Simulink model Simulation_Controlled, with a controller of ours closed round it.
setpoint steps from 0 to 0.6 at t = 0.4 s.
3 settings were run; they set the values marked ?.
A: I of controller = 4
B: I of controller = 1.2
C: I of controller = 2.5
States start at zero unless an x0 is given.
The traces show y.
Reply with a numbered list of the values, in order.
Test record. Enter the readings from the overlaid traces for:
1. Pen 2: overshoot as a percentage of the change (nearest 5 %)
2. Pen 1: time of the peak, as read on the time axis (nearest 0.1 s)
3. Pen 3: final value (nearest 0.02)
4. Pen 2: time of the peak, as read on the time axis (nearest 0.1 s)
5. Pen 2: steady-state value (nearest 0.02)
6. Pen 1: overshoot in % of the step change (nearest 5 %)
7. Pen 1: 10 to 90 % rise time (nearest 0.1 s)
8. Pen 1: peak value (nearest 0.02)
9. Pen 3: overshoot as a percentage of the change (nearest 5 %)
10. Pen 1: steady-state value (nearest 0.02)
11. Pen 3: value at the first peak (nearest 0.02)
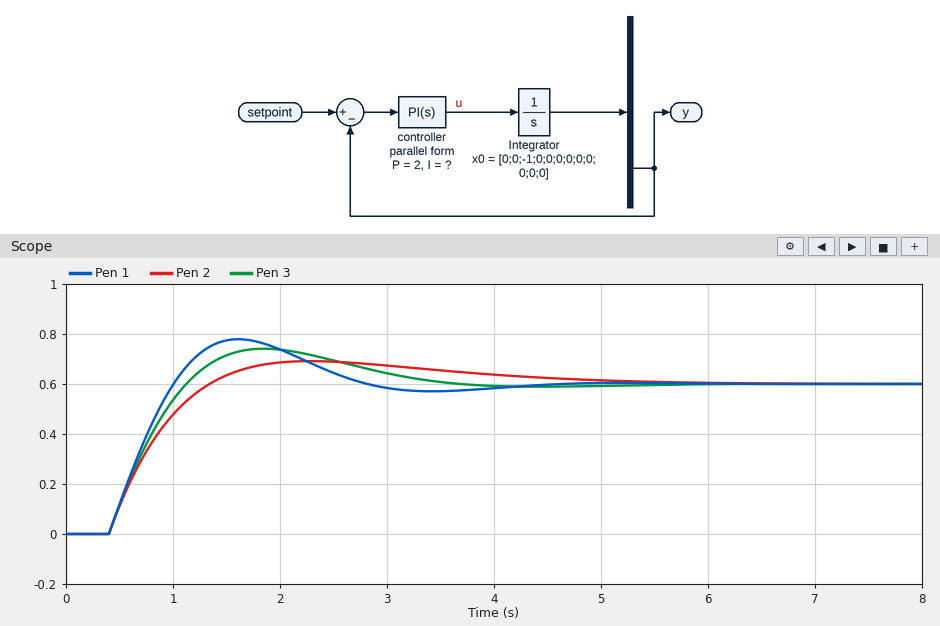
1. 15 %
2. 1.6 s
3. 0.60
4. 2.3 s
5. 0.60
6. 30 %
7. 0.5 s
8. 0.78
9. 25 %
10. 0.60
11. 0.74
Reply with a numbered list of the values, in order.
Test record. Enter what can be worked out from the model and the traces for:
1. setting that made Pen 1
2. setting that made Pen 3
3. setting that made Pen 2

1. A
2. C
3. B
